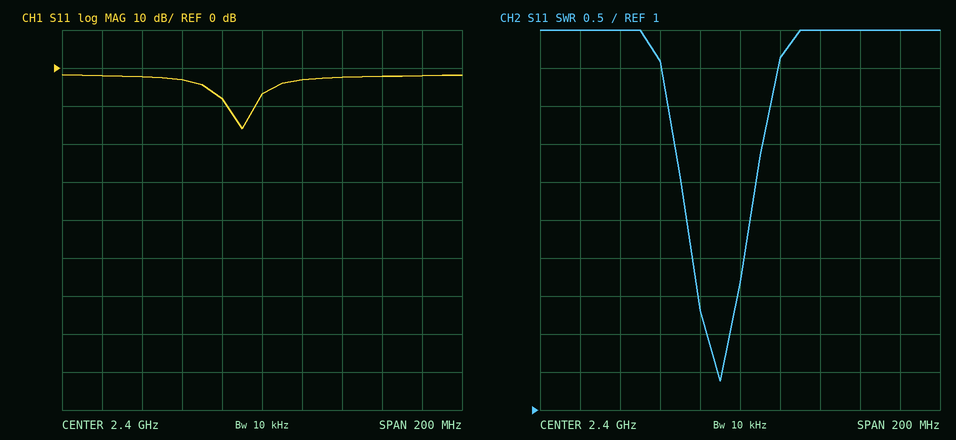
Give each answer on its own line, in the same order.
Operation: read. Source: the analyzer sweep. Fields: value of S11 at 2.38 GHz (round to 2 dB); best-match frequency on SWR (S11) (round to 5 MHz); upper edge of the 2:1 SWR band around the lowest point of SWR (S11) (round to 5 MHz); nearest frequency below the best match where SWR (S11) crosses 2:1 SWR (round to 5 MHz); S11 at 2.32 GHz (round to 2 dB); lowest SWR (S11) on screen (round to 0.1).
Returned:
-8 dB
2.390 GHz
2.395 GHz
2.385 GHz
-2 dB
1.4
